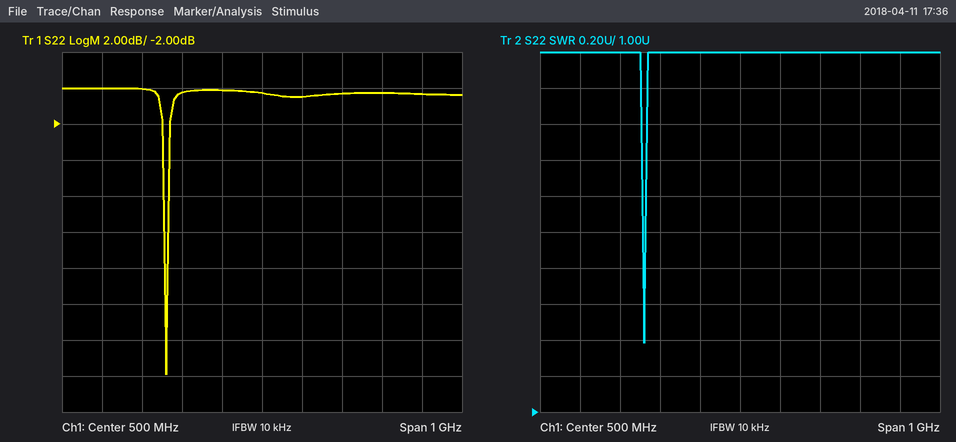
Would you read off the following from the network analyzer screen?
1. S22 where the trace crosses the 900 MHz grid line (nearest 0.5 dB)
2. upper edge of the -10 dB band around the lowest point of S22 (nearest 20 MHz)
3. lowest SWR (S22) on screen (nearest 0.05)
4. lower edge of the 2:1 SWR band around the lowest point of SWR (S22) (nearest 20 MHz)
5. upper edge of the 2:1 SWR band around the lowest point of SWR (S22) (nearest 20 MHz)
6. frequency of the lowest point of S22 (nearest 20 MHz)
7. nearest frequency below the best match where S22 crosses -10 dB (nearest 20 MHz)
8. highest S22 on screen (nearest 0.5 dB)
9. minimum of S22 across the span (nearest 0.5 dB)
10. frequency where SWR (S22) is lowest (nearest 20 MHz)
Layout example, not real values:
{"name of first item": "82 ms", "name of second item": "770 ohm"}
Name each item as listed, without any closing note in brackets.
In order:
{"S22 where the trace crosses the 900 MHz grid line": "-0.5 dB", "upper edge of the -10 dB band around the lowest point of S22": "260 MHz", "lowest SWR (S22) on screen": "1.40", "lower edge of the 2:1 SWR band around the lowest point of SWR (S22)": "260 MHz", "upper edge of the 2:1 SWR band around the lowest point of SWR (S22)": "260 MHz", "frequency of the lowest point of S22": "260 MHz", "nearest frequency below the best match where S22 crosses -10 dB": "260 MHz", "highest S22 on screen": "0.0 dB", "minimum of S22 across the span": "-16.0 dB", "frequency where SWR (S22) is lowest": "260 MHz"}
